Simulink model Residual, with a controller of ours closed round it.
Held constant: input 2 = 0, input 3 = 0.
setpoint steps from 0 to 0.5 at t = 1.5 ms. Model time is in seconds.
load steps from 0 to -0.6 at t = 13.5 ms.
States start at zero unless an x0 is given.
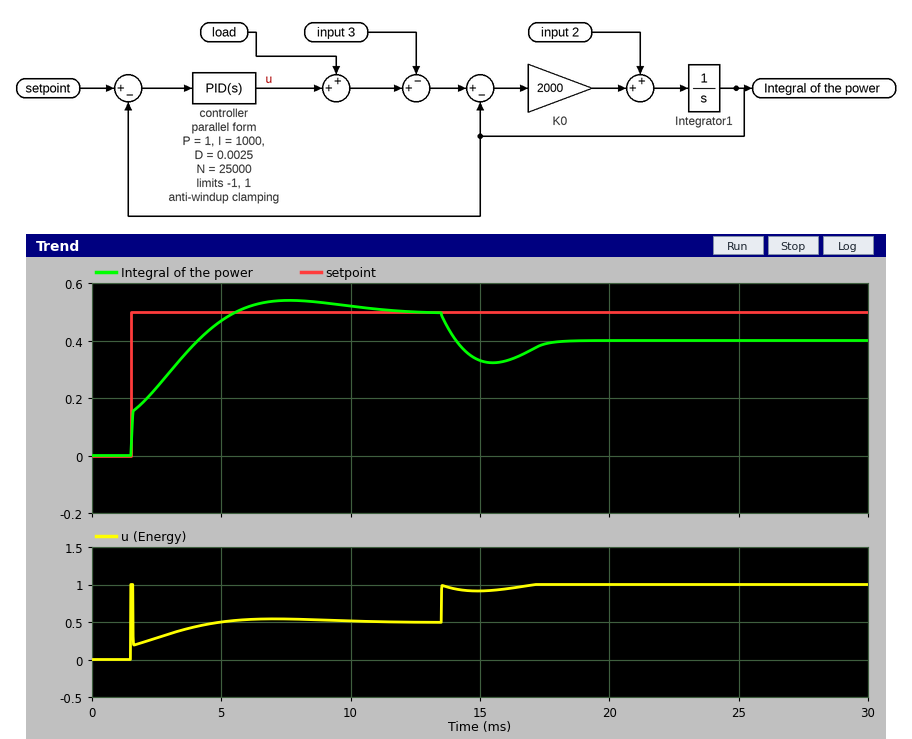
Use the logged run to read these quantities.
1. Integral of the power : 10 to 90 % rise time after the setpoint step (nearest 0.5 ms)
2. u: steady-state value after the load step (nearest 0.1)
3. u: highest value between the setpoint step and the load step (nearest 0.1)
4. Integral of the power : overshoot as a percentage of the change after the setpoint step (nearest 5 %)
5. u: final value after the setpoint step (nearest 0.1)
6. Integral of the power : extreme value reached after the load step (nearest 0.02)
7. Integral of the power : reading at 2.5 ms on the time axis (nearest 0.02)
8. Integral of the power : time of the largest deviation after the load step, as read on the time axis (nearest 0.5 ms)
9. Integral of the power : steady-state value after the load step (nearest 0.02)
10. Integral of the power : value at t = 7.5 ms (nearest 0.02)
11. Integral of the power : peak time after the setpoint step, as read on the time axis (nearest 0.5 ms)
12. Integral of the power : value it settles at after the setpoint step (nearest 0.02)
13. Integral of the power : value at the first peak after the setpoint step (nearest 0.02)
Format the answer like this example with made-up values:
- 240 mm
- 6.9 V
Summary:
- 3.0 ms
- 1.0
- 1.0
- 10 %
- 0.5
- 0.32
- 0.24
- 15.5 ms
- 0.40
- 0.54
- 7.5 ms
- 0.50
- 0.54
